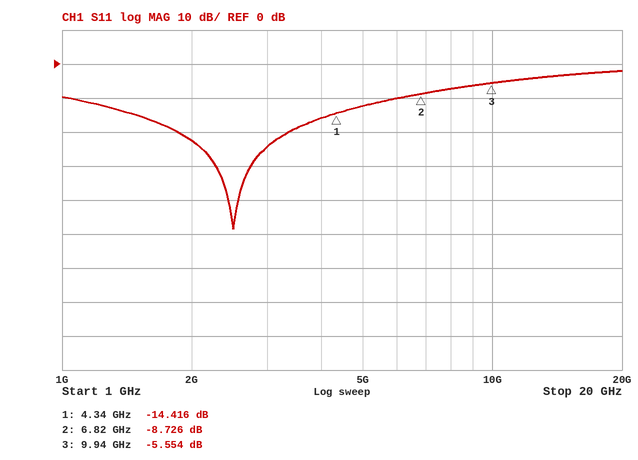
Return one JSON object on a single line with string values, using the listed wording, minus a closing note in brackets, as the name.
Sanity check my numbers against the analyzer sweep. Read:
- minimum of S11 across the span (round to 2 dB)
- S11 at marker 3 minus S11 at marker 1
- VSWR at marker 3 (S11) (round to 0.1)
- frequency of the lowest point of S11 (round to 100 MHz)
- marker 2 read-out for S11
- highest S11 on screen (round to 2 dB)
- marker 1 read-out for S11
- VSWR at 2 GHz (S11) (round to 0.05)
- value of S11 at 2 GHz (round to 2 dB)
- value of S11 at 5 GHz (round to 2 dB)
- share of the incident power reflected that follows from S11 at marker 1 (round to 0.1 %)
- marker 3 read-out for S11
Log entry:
{"minimum of S11 across the span": "-48 dB", "S11 at marker 3 minus S11 at marker 1": "8.862 dB", "VSWR at marker 3 (S11)": "3.2", "frequency of the lowest point of S11": "2.5 GHz", "marker 2 read-out for S11": "-8.726 dB", "highest S11 on screen": "-2 dB", "marker 1 read-out for S11": "-14.416 dB", "VSWR at 2 GHz (S11)": "1.15", "value of S11 at 2 GHz": "-22 dB", "value of S11 at 5 GHz": "-12 dB", "share of the incident power reflected that follows from S11 at marker 1": "3.6 %", "marker 3 read-out for S11": "-5.554 dB"}
